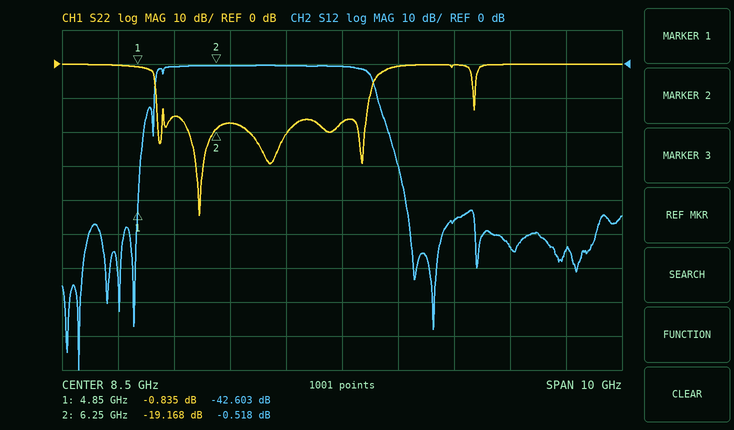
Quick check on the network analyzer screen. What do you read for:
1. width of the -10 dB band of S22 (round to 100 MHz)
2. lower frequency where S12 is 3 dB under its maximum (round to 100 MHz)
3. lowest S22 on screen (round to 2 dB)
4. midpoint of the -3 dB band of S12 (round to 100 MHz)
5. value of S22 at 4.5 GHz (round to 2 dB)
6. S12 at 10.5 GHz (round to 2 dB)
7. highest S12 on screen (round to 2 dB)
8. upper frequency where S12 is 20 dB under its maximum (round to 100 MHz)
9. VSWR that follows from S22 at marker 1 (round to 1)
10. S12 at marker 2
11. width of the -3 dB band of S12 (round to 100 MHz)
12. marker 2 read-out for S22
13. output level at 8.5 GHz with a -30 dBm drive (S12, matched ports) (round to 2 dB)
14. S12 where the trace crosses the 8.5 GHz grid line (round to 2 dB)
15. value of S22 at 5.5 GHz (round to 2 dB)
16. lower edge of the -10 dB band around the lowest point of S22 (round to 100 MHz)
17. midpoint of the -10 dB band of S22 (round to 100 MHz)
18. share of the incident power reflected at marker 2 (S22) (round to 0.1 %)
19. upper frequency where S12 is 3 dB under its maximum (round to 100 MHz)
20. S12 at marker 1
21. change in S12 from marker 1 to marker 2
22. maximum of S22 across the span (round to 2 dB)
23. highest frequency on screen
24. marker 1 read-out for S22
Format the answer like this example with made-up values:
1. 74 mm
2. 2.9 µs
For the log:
1. 3.8 GHz
2. 5.2 GHz
3. -44 dB
4. 7.1 GHz
5. 0 dB
6. -46 dB
7. 0 dB
8. 9.3 GHz
9. 21
10. -0.518 dB
11. 3.8 GHz
12. -19.168 dB
13. -30 dBm
14. 0 dB
15. -16 dB
16. 5.2 GHz
17. 7.1 GHz
18. 1.2 %
19. 9.0 GHz
20. -42.603 dB
21. 42.085 dB
22. 0 dB
23. 13.5 GHz
24. -0.835 dB
